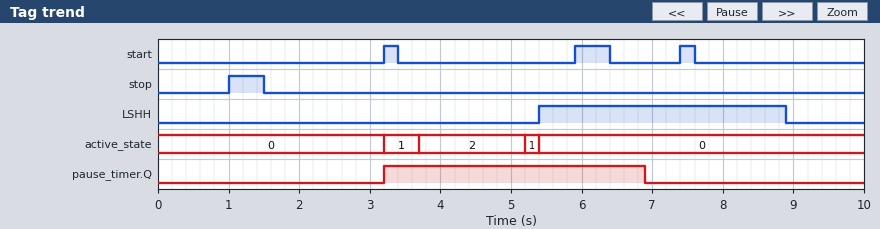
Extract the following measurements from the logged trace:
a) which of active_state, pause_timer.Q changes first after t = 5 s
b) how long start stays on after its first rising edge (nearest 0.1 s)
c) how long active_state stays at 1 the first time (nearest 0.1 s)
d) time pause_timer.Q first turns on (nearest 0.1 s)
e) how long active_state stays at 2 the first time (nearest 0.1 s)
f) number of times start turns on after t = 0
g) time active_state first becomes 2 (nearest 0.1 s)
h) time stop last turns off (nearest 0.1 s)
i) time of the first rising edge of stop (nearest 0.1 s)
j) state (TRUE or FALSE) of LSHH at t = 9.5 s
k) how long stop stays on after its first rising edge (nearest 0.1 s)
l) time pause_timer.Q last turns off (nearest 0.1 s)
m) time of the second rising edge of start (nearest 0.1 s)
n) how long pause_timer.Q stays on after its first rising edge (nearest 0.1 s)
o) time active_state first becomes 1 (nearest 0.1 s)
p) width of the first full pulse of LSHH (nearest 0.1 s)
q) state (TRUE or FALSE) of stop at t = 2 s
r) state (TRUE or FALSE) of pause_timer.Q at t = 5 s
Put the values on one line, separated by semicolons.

active_state; 0.2 s; 0.5 s; 3.2 s; 1.5 s; 3; 3.7 s; 1.5 s; 1.0 s; FALSE; 0.5 s; 6.9 s; 5.9 s; 3.7 s; 3.2 s; 3.5 s; FALSE; TRUE
